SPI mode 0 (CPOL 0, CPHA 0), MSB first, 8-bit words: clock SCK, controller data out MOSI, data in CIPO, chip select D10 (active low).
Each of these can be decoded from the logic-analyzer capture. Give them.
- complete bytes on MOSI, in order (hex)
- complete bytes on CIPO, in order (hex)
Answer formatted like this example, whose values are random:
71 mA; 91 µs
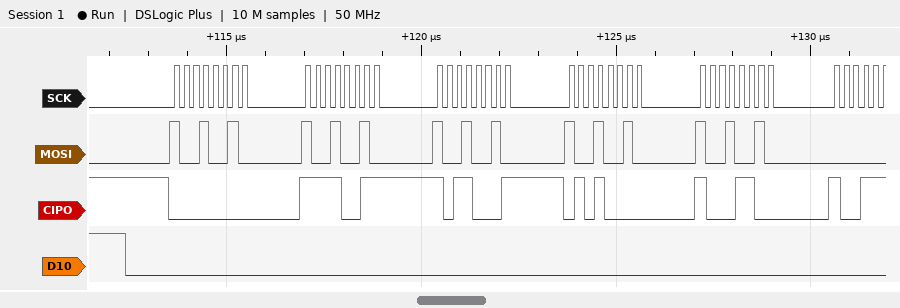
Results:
92 92 92 92 92; 00 F3 B1 50 8C
